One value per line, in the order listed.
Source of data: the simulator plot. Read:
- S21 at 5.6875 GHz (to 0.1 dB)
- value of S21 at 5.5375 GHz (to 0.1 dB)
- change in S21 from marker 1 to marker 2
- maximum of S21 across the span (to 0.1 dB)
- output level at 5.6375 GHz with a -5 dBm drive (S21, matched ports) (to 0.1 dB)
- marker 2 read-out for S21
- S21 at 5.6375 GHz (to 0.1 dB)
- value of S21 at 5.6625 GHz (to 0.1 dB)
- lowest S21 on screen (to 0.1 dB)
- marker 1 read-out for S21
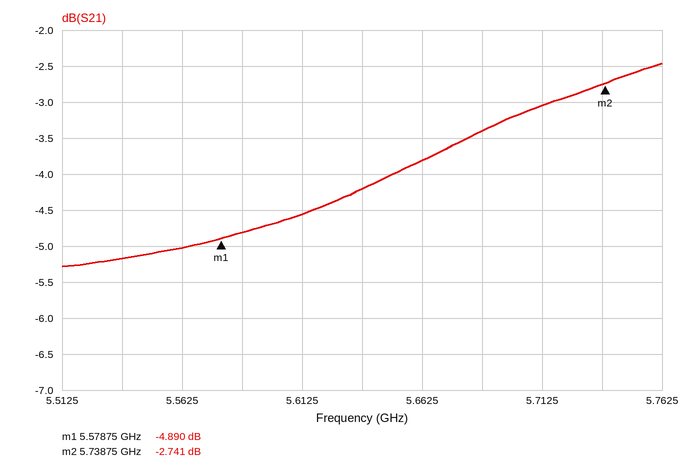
-3.4 dB
-5.2 dB
2.149 dB
-2.5 dB
-9.2 dBm
-2.741 dB
-4.2 dB
-3.8 dB
-5.3 dB
-4.890 dB
